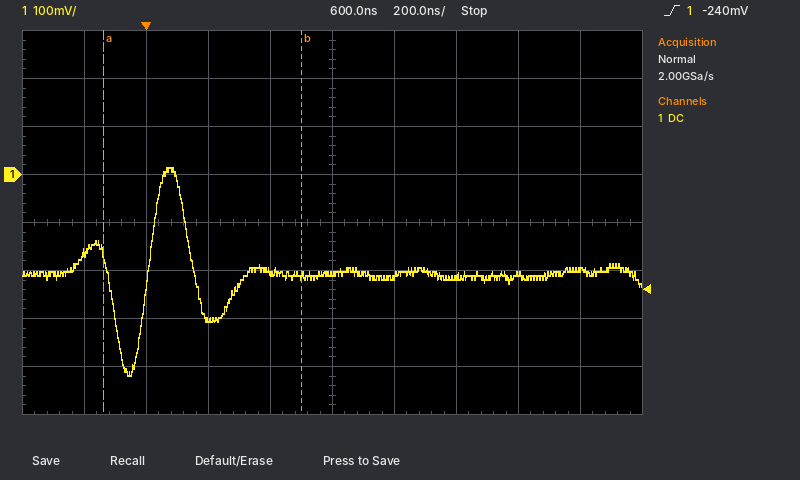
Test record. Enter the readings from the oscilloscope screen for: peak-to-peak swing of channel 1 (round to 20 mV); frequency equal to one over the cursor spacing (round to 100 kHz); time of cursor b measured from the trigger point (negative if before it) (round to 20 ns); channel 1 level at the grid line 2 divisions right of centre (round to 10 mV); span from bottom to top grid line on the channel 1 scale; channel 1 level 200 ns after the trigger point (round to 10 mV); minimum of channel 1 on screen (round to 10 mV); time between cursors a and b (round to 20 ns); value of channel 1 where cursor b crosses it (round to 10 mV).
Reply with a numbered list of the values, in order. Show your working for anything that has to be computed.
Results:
1. 440 mV
2. 1 / 640 ns ≈ 1.6 MHz
3. +500 ns
4. -210 mV
5. 800 mV
6. -300 mV
7. -420 mV
8. 640 ns
9. -210 mV
